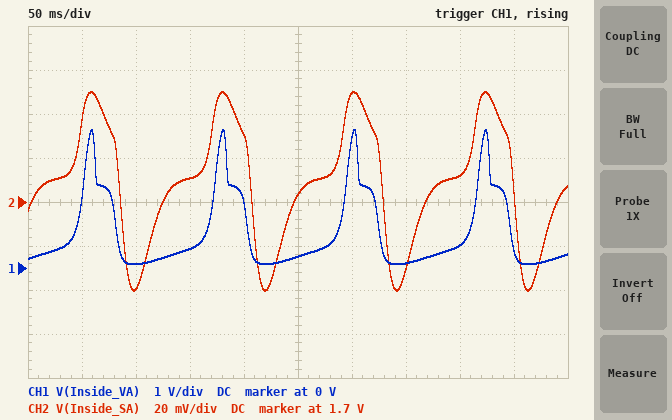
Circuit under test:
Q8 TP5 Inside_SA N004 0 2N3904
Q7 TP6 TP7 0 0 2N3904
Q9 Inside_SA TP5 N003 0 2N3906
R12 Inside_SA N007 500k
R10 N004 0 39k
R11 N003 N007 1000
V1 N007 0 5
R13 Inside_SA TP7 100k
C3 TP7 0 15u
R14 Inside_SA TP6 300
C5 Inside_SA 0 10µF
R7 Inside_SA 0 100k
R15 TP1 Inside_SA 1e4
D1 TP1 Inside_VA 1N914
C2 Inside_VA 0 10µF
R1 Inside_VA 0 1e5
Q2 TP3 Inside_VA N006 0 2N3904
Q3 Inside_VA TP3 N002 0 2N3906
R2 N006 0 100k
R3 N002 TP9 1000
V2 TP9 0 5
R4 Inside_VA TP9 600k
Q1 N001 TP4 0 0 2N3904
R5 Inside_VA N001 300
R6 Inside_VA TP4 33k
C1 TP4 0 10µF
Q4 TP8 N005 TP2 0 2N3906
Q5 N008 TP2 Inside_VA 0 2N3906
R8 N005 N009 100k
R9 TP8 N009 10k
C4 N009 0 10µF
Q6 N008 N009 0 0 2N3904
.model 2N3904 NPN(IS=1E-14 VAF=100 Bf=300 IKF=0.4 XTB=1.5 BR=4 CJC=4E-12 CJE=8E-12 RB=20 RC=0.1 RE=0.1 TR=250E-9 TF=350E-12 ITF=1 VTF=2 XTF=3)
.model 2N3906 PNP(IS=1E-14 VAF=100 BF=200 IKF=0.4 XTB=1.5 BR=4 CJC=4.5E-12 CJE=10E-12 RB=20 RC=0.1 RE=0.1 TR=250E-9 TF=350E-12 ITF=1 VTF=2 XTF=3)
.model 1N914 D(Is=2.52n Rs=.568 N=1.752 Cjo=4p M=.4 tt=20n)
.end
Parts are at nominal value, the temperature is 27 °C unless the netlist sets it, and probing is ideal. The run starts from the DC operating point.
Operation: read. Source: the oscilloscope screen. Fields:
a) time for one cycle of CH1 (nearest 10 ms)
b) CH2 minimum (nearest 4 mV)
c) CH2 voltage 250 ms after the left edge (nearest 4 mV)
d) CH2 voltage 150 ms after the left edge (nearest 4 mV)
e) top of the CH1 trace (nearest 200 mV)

120 ms
1.660 V
1.704 V
1.712 V
3.2 V
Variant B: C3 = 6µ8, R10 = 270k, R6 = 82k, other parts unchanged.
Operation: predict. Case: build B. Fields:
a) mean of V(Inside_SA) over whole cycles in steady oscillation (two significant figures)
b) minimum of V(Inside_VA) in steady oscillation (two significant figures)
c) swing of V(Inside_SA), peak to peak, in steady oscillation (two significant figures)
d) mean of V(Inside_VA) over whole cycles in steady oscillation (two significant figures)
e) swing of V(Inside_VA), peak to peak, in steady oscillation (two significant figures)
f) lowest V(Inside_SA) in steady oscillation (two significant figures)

620 mV
18 mV
4.5 V
680 mV
3.4 V
21 mV
